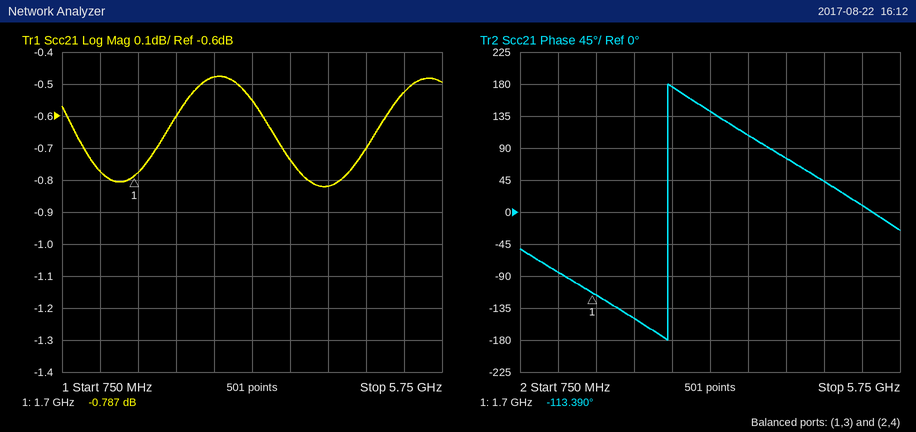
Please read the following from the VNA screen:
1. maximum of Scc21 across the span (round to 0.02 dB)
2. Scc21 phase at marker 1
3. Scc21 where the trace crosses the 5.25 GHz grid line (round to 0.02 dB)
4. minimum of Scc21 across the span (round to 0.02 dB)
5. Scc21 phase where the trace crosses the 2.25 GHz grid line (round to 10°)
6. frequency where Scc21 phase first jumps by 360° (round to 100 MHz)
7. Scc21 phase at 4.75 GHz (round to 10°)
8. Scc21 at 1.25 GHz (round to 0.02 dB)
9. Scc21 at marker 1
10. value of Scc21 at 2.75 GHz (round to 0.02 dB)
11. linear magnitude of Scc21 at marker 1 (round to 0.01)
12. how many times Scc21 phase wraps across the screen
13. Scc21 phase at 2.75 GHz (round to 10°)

-0.48 dB
-113.390°
-0.52 dB
-0.82 dB
-150°
2.7 GHz
40°
-0.78 dB
-0.787 dB
-0.48 dB
0.91
1
180°
